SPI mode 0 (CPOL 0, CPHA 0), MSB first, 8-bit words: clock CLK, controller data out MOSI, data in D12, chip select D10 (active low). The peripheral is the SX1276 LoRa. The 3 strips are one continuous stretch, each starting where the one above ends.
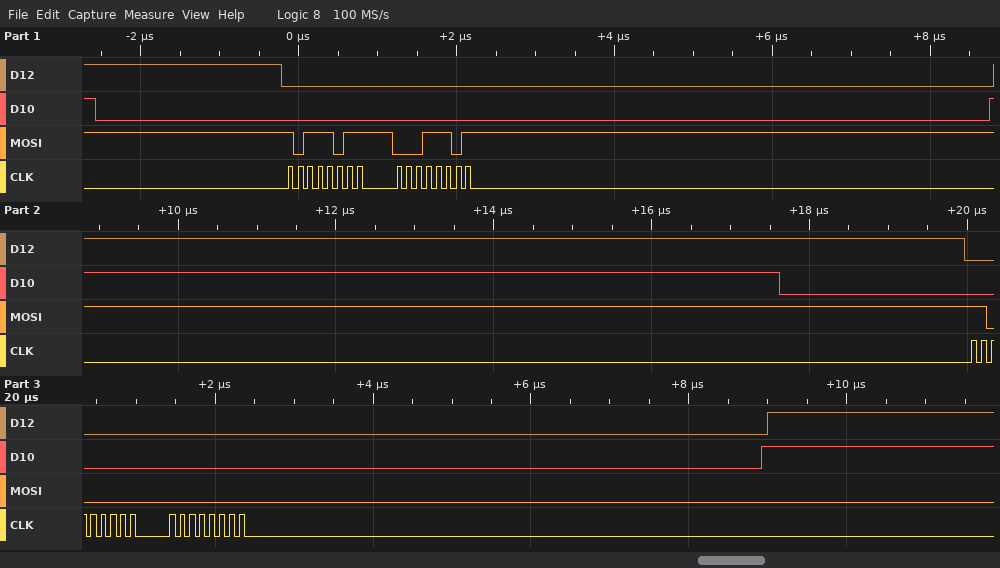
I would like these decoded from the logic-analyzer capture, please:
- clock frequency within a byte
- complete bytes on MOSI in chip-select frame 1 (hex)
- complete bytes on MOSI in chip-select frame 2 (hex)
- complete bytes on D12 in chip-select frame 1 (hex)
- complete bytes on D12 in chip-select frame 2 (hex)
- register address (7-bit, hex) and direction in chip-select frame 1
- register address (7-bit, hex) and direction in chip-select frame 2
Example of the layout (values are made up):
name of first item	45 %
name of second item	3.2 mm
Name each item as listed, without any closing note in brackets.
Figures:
clock frequency within a byte	8 MHz
complete bytes on MOSI in chip-select frame 1	BB 1D
complete bytes on MOSI in chip-select frame 2	C0 00
complete bytes on D12 in chip-select frame 1	00 00
complete bytes on D12 in chip-select frame 2	00 00
register address (7-bit, hex) and direction in chip-select frame 1	0x3B write
register address (7-bit, hex) and direction in chip-select frame 2	0x40 write
